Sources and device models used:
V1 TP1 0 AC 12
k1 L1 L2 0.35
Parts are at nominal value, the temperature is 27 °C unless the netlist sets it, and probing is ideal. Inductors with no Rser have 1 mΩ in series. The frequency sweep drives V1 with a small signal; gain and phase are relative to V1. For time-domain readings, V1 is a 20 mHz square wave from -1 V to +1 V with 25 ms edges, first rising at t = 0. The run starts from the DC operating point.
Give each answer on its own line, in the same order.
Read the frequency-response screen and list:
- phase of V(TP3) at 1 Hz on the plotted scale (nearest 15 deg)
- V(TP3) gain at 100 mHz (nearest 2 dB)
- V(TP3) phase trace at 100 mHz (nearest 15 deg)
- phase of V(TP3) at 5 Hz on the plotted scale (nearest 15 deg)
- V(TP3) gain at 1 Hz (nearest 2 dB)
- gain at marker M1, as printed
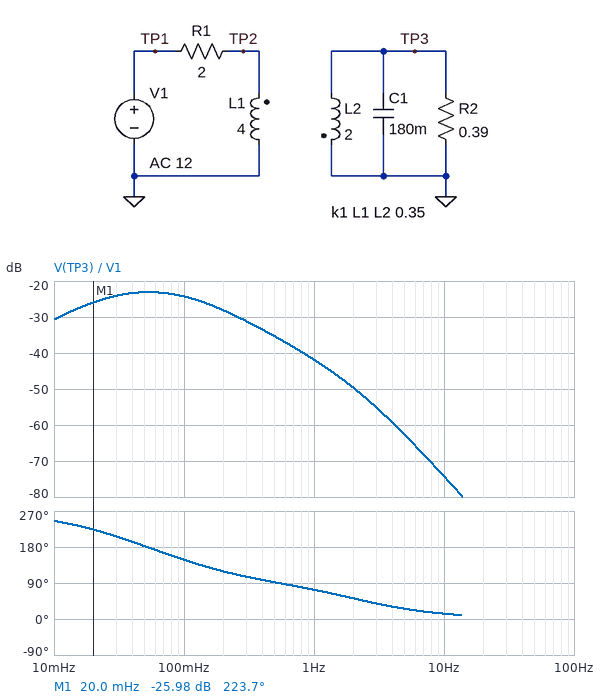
75 deg
-24 dB
150 deg
30 deg
-42 dB
-25.98 dB
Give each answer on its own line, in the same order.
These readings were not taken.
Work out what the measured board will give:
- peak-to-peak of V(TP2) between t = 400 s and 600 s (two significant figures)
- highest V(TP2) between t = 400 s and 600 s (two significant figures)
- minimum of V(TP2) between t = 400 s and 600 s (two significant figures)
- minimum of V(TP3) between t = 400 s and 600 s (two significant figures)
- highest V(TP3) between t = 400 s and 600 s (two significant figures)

4.0 V
2.0 V
-2.0 V
-110 mV
110 mV
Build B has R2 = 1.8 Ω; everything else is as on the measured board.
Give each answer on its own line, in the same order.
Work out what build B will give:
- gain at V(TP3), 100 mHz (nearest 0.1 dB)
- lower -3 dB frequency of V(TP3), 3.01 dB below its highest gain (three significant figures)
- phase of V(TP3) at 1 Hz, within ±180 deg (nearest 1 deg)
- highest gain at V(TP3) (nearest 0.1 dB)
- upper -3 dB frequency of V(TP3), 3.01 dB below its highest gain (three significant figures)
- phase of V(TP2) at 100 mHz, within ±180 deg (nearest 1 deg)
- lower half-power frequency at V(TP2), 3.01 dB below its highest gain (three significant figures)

-15.3 dB
50.0 mHz
33 deg
-15.0 dB
300 mHz
38 deg
87.4 mHz
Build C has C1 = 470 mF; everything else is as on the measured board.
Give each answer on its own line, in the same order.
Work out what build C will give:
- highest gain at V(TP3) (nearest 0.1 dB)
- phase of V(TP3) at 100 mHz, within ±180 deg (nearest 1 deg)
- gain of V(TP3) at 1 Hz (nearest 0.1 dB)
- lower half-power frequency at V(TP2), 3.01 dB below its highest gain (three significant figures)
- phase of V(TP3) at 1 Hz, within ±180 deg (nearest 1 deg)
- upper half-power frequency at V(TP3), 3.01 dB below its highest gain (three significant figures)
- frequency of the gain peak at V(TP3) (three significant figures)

-23.0 dB
144 deg
-44.7 dB
93.8 mHz
47 deg
145 mHz
54.0 mHz
